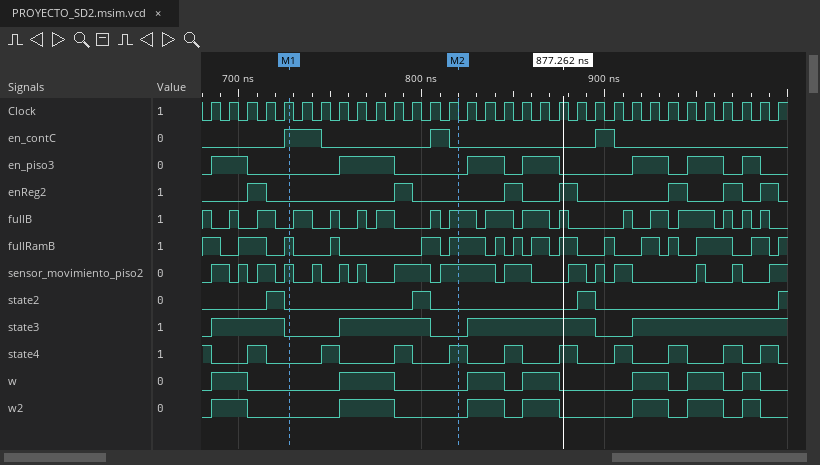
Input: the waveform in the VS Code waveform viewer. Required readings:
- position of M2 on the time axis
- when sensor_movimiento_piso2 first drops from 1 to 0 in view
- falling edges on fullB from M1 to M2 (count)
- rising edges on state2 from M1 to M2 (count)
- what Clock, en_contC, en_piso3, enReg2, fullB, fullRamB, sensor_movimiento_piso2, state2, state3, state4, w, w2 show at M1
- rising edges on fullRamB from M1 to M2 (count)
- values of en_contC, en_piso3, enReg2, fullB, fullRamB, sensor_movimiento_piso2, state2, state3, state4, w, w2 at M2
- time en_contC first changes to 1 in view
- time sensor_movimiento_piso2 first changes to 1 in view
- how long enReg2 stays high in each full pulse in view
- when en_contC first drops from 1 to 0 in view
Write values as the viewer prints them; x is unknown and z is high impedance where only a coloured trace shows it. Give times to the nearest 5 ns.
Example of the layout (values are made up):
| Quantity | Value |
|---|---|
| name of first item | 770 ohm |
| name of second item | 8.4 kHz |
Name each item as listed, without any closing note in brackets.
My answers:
| Quantity | Value |
|---|---|
| position of M2 on the time axis | 820 ns |
| when sensor_movimiento_piso2 first drops from 1 to 0 in view | 695 ns |
| falling edges on fullB from M1 to M2 | 5 |
| rising edges on state2 from M1 to M2 | 1 |
| what Clock, en_contC, en_piso3, enReg2, fullB, fullRamB, sensor_movimiento_piso2, state2, state3, state4, w, w2 show at M1 | Clock=1, en_contC=1, en_piso3=0, enReg2=0, fullB=0, fullRamB=1, sensor_movimiento_piso2=1, state2=0, state3=0, state4=0, w=0, w2=0 |
| rising edges on fullRamB from M1 to M2 | 3 |
| values of en_contC, en_piso3, enReg2, fullB, fullRamB, sensor_movimiento_piso2, state2, state3, state4, w, w2 at M2 | en_contC=0, en_piso3=0, enReg2=0, fullB=1, fullRamB=1, sensor_movimiento_piso2=1, state2=0, state3=0, state4=1, w=0, w2=0 |
| time en_contC first changes to 1 in view | 725 ns |
| time sensor_movimiento_piso2 first changes to 1 in view | 685 ns |
| how long enReg2 stays high in each full pulse in view | 10 ns, 10 ns, 10 ns, 10 ns, 10 ns, 10 ns, 10 ns |
| when en_contC first drops from 1 to 0 in view | 745 ns |
